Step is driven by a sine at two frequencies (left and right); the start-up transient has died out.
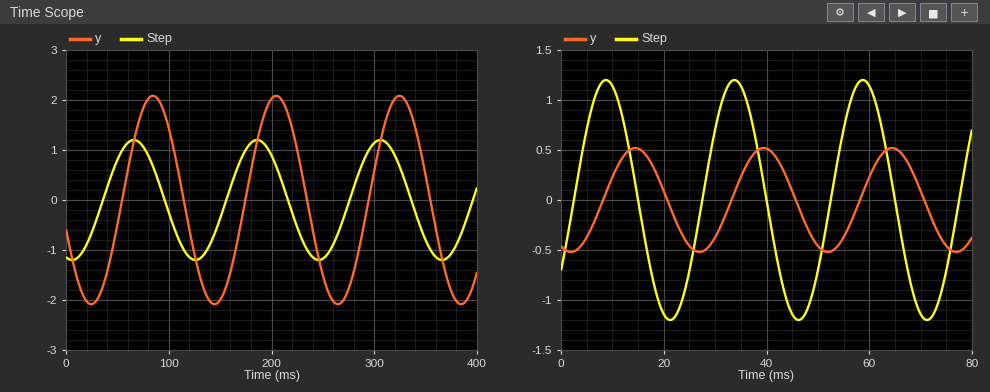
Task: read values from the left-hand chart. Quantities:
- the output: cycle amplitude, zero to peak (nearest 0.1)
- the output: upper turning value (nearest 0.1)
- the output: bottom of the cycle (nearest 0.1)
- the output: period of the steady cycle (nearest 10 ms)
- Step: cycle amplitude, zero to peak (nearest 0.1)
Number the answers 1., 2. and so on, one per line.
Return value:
1. 2.1
2. 2.1
3. -2.1
4. 120 ms
5. 1.2
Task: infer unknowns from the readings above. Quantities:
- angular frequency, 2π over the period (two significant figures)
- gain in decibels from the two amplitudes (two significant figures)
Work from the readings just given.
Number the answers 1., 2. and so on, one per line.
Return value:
1. 0.052 rad/ms
2. 4.9 dB
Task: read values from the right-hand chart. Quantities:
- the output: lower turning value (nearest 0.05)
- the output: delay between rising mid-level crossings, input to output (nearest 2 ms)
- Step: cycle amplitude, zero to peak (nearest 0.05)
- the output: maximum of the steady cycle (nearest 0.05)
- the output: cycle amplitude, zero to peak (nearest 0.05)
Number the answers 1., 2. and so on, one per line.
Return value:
1. -0.50
2. 6 ms
3. 1.20
4. 0.50
5. 0.50
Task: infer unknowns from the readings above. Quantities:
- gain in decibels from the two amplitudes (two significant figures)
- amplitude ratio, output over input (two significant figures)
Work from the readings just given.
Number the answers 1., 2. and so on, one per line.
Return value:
1. -7.6 dB
2. 0.42
